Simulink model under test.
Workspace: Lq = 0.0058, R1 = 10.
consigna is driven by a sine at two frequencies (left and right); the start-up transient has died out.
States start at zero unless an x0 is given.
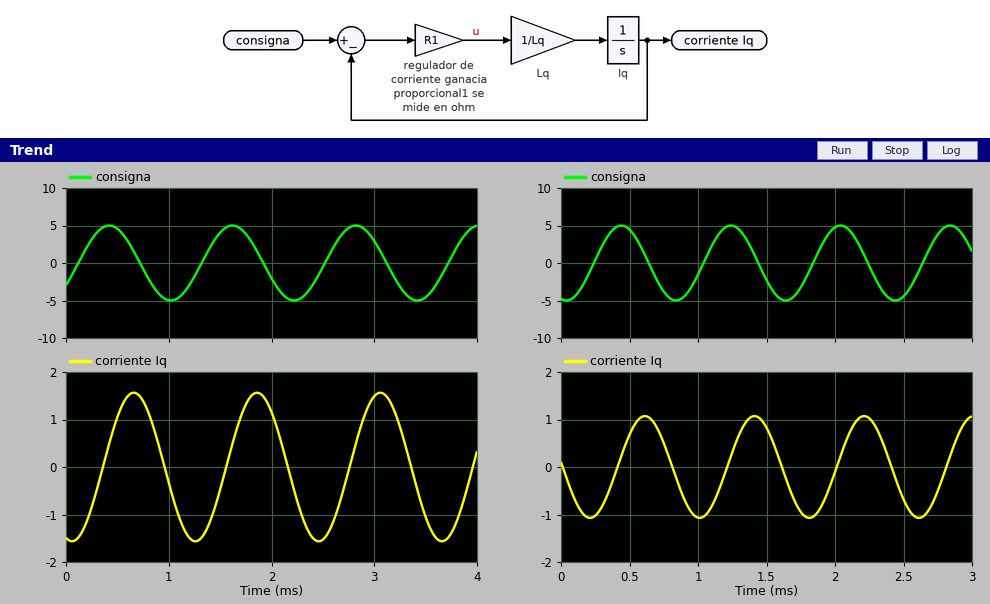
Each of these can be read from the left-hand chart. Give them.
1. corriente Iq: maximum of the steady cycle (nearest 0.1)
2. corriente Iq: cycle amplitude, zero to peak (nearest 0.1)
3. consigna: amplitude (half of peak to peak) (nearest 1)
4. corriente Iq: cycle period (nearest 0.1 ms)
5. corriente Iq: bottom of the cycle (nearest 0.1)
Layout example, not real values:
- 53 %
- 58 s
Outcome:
- 1.6
- 1.6
- 5
- 1.2 ms
- -1.6
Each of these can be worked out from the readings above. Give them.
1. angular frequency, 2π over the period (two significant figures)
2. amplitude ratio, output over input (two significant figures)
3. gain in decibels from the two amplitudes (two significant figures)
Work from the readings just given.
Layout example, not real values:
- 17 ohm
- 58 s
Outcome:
- 5.2 rad/ms
- 0.32
- -9.9 dB
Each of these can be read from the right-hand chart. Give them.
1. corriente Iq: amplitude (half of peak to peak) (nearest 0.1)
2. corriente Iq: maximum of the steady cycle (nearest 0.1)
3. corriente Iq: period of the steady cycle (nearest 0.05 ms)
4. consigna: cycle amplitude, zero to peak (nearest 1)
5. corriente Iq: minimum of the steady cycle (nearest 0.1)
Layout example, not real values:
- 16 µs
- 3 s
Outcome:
- 1.1
- 1.1
- 0.80 ms
- 5
- -1.1
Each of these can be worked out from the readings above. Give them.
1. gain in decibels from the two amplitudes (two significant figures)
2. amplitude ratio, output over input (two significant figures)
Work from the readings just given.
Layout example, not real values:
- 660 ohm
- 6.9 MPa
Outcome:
- -13 dB
- 0.22
